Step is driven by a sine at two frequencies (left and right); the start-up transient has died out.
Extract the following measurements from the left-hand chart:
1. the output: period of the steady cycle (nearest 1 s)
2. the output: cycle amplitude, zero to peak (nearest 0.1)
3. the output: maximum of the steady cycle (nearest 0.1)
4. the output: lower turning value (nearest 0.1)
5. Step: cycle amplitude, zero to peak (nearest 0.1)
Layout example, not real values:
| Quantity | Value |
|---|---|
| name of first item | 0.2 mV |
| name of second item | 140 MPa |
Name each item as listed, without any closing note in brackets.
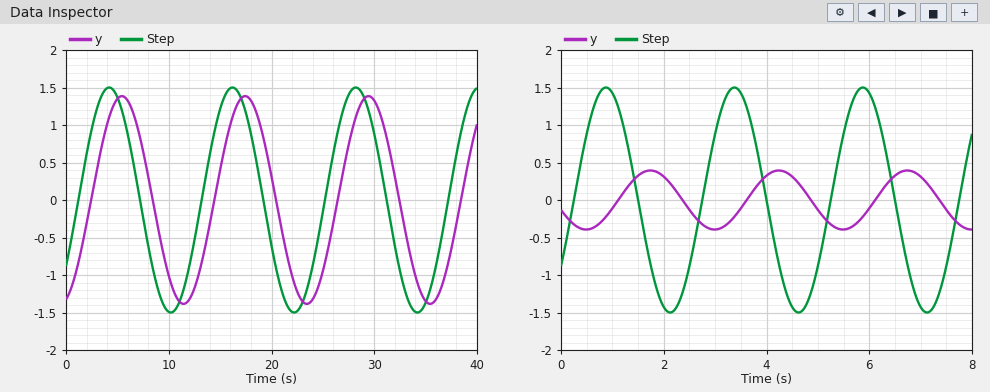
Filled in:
| Quantity | Value |
|---|---|
| the output: period of the steady cycle | 12 s |
| the output: cycle amplitude, zero to peak | 1.4 |
| the output: maximum of the steady cycle | 1.4 |
| the output: lower turning value | -1.4 |
| Step: cycle amplitude, zero to peak | 1.5 |
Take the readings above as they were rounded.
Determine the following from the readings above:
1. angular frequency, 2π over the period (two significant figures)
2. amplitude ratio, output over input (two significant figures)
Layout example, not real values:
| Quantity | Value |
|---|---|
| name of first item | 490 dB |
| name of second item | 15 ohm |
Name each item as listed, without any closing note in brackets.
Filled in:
| Quantity | Value |
|---|---|
| angular frequency, 2π over the period | 0.52 rad/s |
| amplitude ratio, output over input | 0.93 |
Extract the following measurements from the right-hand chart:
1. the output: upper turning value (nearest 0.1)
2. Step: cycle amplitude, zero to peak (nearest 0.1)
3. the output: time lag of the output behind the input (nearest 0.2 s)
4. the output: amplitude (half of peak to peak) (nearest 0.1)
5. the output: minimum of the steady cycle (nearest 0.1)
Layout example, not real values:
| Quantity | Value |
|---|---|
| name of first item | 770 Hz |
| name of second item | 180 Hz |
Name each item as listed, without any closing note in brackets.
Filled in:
| Quantity | Value |
|---|---|
| the output: upper turning value | 0.4 |
| Step: cycle amplitude, zero to peak | 1.5 |
| the output: time lag of the output behind the input | 0.8 s |
| the output: amplitude (half of peak to peak) | 0.4 |
| the output: minimum of the steady cycle | -0.4 |
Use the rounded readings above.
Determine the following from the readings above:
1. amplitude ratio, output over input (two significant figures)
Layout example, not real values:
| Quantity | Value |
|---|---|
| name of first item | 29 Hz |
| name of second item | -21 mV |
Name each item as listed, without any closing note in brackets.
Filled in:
| Quantity | Value |
|---|---|
| amplitude ratio, output over input | 0.27 |
